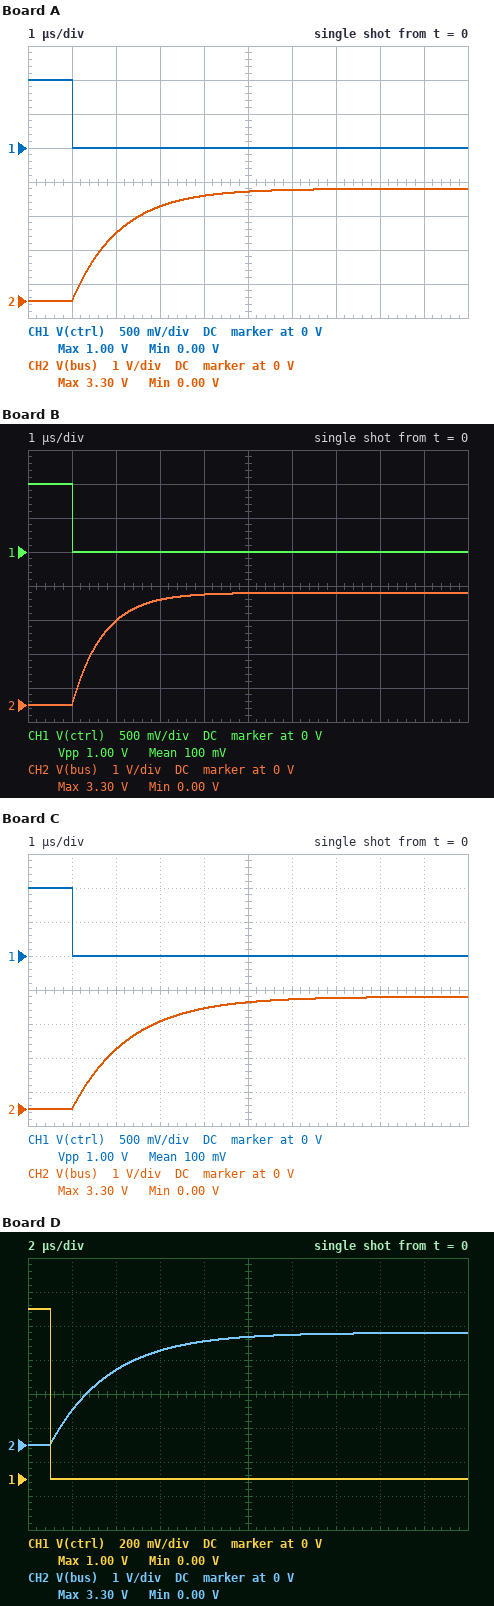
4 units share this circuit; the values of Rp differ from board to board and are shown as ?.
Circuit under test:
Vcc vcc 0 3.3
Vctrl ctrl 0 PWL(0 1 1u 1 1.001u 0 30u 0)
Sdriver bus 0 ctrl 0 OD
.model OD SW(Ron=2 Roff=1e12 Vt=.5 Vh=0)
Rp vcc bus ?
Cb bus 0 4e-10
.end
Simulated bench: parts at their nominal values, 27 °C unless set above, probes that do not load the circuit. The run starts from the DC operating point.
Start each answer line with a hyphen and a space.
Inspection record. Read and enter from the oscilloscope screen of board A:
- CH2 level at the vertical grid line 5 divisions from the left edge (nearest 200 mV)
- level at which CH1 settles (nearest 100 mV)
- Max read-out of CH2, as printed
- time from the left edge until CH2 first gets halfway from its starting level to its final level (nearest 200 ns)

- 3.2 V
- 0 V
- 3.30 V
- 1.8 µs
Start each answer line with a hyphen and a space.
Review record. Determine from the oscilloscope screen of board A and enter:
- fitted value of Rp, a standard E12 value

- 2.7 kΩ
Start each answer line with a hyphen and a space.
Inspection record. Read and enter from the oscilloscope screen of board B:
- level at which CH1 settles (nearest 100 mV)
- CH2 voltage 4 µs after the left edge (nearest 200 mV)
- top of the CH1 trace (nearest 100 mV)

- 0 V
- 3.2 V
- 1.0 V
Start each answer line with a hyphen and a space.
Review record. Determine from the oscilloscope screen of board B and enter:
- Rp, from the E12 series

- 1.8 kΩ
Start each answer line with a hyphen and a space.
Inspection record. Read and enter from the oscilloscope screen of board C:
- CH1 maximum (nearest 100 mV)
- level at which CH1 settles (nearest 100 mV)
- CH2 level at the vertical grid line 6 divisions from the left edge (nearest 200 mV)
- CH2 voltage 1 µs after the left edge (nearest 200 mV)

- 1.0 V
- 0 V
- 3.2 V
- 0 V
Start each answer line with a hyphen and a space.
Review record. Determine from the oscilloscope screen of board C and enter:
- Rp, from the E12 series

- 3.3 kΩ
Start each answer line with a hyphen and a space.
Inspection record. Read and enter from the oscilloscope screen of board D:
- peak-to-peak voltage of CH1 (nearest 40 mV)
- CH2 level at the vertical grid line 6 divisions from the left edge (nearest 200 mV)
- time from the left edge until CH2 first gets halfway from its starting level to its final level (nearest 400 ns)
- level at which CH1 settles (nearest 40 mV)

- 1.00 V
- 3.2 V
- 2.8 µs
- 0 V
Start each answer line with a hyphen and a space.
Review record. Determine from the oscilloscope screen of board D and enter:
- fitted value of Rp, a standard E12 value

- 6.8 kΩ
